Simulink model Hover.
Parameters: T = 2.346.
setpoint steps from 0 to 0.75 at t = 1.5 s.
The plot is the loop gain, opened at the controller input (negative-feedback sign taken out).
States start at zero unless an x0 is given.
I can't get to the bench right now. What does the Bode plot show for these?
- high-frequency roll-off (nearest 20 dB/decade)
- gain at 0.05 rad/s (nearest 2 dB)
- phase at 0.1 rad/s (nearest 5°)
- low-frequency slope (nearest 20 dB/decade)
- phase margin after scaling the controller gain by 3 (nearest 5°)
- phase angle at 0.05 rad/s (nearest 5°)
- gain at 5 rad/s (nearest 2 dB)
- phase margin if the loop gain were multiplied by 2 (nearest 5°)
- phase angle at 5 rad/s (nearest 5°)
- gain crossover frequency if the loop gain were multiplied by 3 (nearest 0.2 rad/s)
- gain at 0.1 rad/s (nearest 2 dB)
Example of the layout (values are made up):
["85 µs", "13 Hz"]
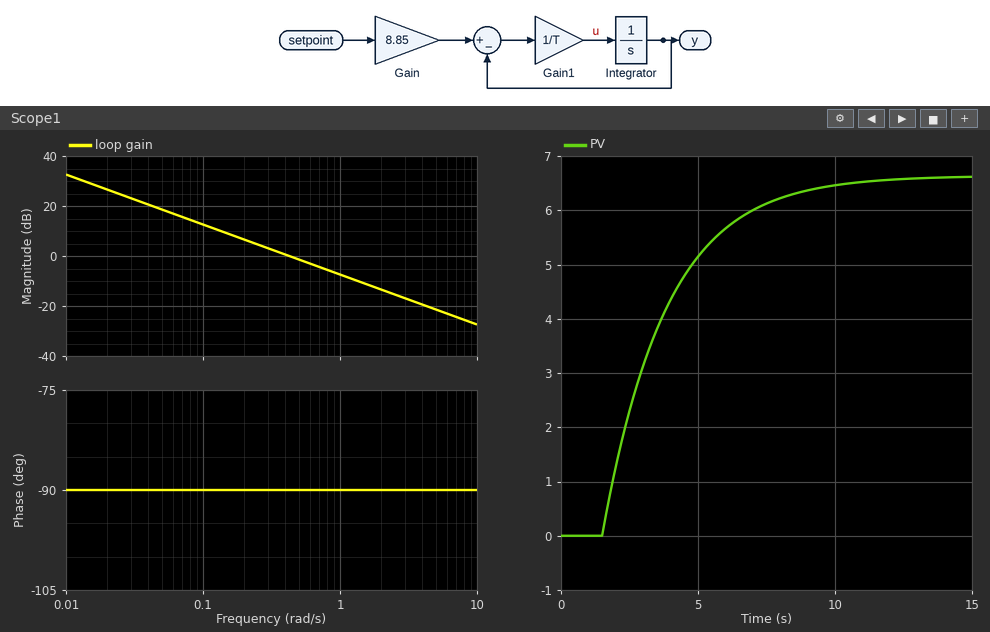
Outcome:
["-20 dB/decade", "18 dB", "-90°", "-20 dB/decade", "90°", "-90°", "-22 dB", "90°", "-90°", "1.2 rad/s", "12 dB"]
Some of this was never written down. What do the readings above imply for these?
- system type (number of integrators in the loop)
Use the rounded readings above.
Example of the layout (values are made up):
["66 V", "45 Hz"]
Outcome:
["1"]
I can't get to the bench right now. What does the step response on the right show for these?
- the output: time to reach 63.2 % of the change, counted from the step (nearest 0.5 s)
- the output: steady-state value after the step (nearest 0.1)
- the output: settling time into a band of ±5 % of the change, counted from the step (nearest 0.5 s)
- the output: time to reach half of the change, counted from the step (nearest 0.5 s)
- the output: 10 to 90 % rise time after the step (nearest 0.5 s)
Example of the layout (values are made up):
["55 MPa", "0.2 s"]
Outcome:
["2.5 s", "6.6", "7.0 s", "1.5 s", "5.0 s"]
